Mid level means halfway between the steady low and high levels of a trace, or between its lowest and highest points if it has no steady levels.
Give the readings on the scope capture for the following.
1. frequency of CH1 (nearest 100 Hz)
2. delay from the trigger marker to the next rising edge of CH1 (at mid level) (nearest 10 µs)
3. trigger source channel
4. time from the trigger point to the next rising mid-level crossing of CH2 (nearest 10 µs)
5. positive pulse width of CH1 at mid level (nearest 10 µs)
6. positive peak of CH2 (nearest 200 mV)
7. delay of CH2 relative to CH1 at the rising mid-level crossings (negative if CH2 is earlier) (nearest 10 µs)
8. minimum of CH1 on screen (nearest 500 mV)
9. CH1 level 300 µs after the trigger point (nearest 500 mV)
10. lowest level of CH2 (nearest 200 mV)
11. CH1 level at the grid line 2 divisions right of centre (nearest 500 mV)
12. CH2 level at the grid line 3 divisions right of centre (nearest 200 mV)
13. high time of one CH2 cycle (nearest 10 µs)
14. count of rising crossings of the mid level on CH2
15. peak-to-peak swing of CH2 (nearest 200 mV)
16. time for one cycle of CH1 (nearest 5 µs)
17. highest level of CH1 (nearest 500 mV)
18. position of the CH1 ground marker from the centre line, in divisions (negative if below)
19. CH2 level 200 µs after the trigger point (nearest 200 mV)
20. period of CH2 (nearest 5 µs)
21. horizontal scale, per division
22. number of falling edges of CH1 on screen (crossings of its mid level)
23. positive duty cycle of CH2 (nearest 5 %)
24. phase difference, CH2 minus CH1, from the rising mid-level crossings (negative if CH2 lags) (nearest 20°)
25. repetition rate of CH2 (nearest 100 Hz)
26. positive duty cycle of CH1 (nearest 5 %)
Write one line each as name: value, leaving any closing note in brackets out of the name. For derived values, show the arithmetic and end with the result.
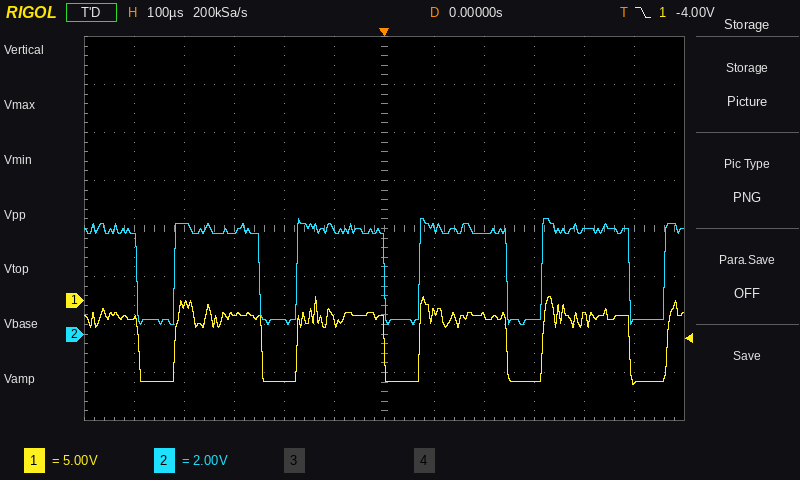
frequency of CH1: 1 / 245 µs ≈ 4.1 kHz
delay from the trigger marker to the next rising edge of CH1 (at mid level): 70 µs
trigger source channel: CH1
time from the trigger point to the next rising mid-level crossing of CH2: 70 µs
positive pulse width of CH1 at mid level: 170 µs
positive peak of CH2: 4.8 V
delay of CH2 relative to CH1 at the rising mid-level crossings (negative if CH2 is earlier): 0 µs
minimum of CH1 on screen: -9.0 V
CH1 level 300 µs after the trigger point: -8.5 V
lowest level of CH2: 400 mV
CH1 level at the grid line 2 divisions right of centre: -1.5 V
CH2 level at the grid line 3 divisions right of centre: 600 mV
high time of one CH2 cycle: 170 µs
count of rising crossings of the mid level on CH2: 5
peak-to-peak swing of CH2: 4.8 V − (400 mV) = 4.4 V
time for one cycle of CH1: 245 µs
highest level of CH1: 500 mV
position of the CH1 ground marker from the centre line, in divisions: -1.5 div
CH2 level 200 µs after the trigger point: 4.2 V
period of CH2: 245 µs
horizontal scale, per division: 100 µs
number of falling edges of CH1 on screen: 5
positive duty cycle of CH2: 170 µs / 245 µs ≈ 69.4 %, so 70 % to the nearest 5 %
phase difference, CH2 minus CH1, from the rising mid-level crossings (negative if CH2 lags): −360° × (0 µs) / 245 µs ≈ 0°
repetition rate of CH2: 1 / 245 µs ≈ 4.1 kHz
positive duty cycle of CH1: 170 µs / 245 µs ≈ 69.4 %, so 70 % to the nearest 5 %
